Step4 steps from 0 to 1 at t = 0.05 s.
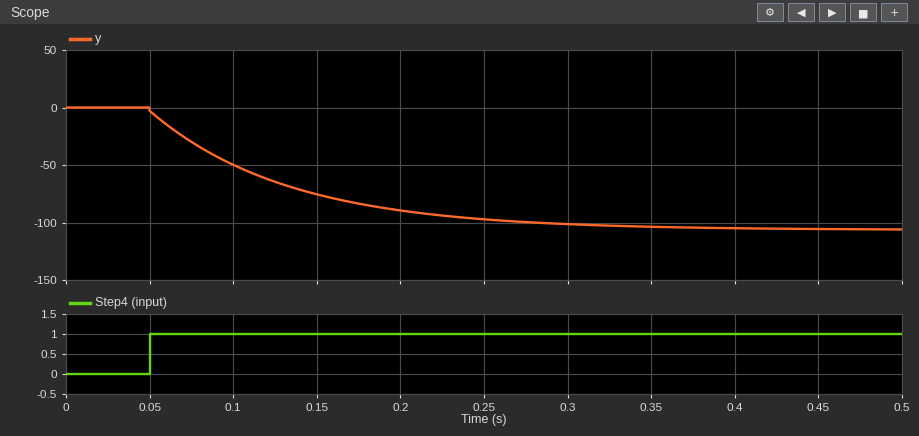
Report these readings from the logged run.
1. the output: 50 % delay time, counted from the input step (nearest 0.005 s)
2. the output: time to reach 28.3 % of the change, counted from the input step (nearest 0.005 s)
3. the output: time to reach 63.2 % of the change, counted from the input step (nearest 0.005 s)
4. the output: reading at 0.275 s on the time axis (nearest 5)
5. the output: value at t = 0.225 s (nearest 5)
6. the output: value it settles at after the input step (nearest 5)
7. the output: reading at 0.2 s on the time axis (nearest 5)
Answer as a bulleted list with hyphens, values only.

- 0.055 s
- 0.025 s
- 0.080 s
- -100
- -95
- -105
- -90
